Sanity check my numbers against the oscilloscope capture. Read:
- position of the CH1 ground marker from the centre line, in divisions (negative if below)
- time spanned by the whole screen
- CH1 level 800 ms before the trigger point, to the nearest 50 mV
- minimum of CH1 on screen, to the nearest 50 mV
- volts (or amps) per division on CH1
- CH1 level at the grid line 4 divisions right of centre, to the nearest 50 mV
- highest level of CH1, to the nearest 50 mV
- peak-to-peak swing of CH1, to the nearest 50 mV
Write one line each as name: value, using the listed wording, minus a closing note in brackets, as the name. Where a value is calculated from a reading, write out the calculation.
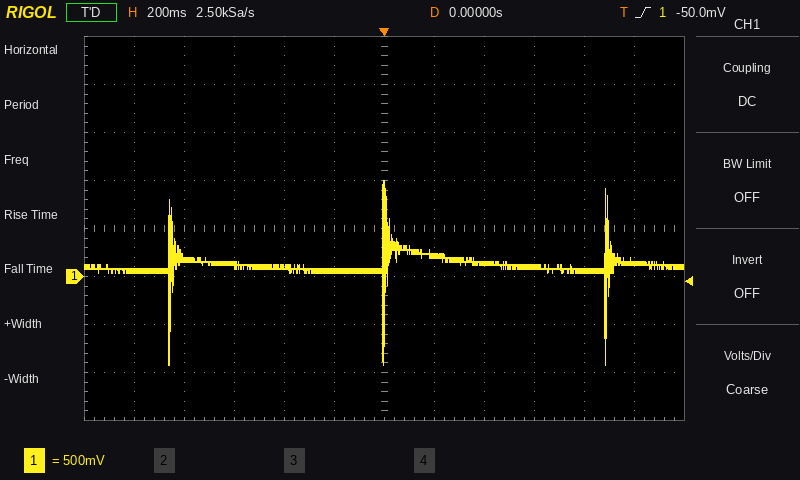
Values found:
position of the CH1 ground marker from the centre line, in divisions: -1.0 div
time spanned by the whole screen: 2.4 s
CH1 level 800 ms before the trigger point, to the nearest 50 mV: 200 mV
minimum of CH1 on screen, to the nearest 50 mV: -900 mV
volts (or amps) per division on CH1: 500 mV
CH1 level at the grid line 4 divisions right of centre, to the nearest 50 mV: 50 mV
highest level of CH1, to the nearest 50 mV: 1.00 V
peak-to-peak swing of CH1, to the nearest 50 mV: 1.00 V − (-900 mV) = 1.90 V
